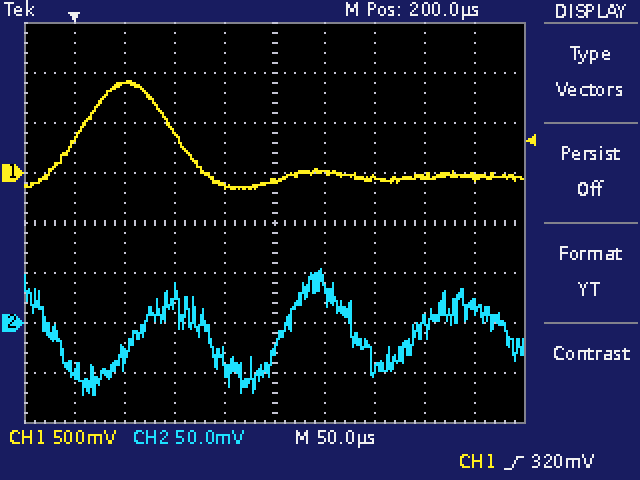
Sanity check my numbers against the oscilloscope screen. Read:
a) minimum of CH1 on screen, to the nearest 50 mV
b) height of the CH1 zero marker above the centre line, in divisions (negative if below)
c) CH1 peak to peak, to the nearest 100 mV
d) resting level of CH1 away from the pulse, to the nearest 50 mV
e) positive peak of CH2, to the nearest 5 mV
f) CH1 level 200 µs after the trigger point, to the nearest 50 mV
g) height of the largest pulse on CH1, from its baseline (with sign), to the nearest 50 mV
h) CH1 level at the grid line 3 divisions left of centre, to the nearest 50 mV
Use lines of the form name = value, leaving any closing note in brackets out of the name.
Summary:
minimum of CH1 on screen, to the nearest 50 mV = -150 mV
height of the CH1 zero marker above the centre line, in divisions = +1.0 div
CH1 peak to peak, to the nearest 100 mV = 1.10 V
resting level of CH1 away from the pulse, to the nearest 50 mV = -50 mV
positive peak of CH2, to the nearest 5 mV = 55 mV
CH1 level 200 µs after the trigger point, to the nearest 50 mV = -100 mV
height of the largest pulse on CH1, from its baseline (with sign), to the nearest 50 mV = +950 mV
CH1 level at the grid line 3 divisions left of centre, to the nearest 50 mV = 900 mV
